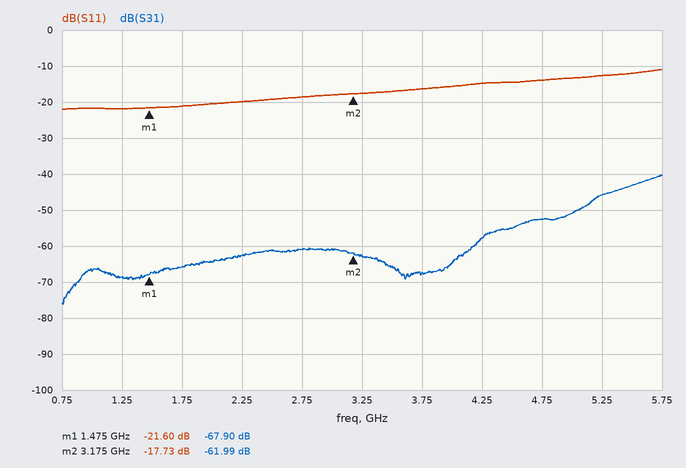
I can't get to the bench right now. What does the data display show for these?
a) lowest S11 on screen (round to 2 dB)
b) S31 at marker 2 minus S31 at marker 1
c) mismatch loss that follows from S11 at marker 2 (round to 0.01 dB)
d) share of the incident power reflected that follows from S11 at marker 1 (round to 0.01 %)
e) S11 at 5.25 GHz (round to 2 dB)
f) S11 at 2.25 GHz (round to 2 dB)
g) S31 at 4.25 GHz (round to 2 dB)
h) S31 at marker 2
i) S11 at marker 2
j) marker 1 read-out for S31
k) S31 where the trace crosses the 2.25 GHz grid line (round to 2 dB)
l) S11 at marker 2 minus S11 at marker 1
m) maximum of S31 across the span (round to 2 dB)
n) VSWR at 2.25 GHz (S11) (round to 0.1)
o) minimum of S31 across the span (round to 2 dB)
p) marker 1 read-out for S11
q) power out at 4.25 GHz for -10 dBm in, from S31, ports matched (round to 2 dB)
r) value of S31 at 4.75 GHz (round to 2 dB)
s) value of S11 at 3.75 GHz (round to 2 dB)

-22 dB
5.91 dB
0.07 dB
0.69 %
-12 dB
-20 dB
-58 dB
-61.99 dB
-17.73 dB
-67.90 dB
-62 dB
3.87 dB
-40 dB
1.2
-76 dB
-21.60 dB
-68 dBm
-52 dB
-16 dB
